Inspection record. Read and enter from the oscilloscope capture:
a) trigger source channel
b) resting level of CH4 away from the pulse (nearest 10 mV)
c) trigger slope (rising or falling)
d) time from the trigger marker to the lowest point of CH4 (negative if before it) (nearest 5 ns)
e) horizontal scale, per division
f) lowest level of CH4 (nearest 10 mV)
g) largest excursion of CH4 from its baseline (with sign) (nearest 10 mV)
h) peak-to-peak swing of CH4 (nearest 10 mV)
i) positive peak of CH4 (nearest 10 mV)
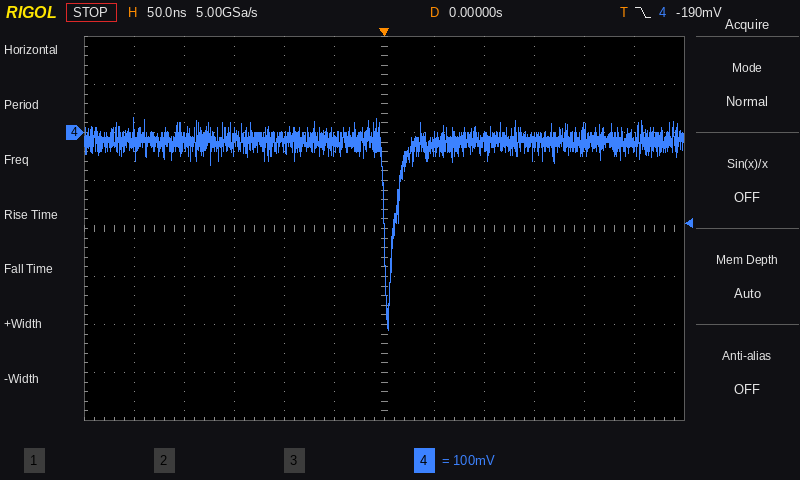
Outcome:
CH4
-20 mV
falling
+5 ns
50 ns
-410 mV
-390 mV
440 mV
30 mV
